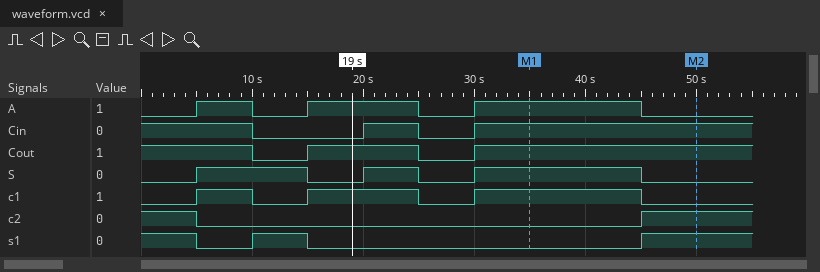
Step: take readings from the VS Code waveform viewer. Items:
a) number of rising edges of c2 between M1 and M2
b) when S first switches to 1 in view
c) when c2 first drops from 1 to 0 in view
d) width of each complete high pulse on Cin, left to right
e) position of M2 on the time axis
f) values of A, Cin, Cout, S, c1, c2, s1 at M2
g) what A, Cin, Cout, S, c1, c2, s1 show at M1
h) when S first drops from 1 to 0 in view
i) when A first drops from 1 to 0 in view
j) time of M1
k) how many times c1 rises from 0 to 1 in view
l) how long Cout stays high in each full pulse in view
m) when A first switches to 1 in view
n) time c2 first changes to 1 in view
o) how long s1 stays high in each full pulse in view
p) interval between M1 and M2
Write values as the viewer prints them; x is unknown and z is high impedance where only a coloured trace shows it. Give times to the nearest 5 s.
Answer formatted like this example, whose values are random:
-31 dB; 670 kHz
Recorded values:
1; 5 s; 5 s; 5 s; 50 s; A=0, Cin=1, Cout=1, S=0, c1=0, c2=1, s1=1; A=1, Cin=1, Cout=1, S=1, c1=1, c2=0, s1=0; 15 s; 10 s; 35 s; 3; 10 s; 5 s; 45 s; 5 s; 15 s
